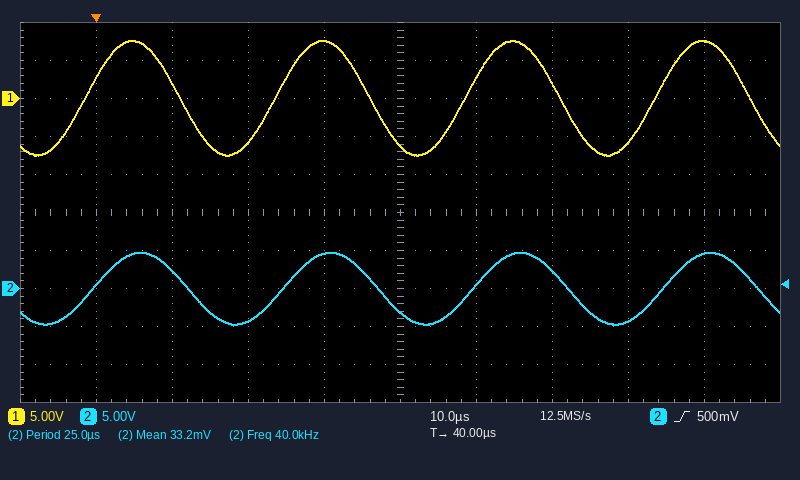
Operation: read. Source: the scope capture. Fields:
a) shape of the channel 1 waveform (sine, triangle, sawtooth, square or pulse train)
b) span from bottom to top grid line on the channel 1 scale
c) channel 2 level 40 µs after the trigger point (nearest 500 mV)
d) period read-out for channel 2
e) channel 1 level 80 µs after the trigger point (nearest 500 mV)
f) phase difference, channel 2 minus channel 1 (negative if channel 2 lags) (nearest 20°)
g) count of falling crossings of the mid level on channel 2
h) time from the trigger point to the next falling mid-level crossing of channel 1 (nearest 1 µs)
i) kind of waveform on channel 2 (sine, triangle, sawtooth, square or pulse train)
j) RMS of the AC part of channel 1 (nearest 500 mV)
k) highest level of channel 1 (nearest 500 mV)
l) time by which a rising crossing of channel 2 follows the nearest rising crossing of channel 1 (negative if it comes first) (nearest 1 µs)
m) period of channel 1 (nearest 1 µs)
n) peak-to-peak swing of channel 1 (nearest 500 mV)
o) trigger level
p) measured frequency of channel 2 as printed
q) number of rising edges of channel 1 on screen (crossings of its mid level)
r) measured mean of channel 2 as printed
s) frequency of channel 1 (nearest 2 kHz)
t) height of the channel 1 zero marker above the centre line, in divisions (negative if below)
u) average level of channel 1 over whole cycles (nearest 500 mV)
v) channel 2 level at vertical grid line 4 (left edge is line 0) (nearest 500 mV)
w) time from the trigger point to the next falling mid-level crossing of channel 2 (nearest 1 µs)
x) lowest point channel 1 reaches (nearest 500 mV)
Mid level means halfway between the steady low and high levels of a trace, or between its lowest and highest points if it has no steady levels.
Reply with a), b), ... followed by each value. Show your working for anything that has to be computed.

a) sine
b) 50 V
c) -3.0 V
d) 25.0 µs
e) 7.5 V
f) −360° × (+1 µs) / 25 µs ≈ -14.4°, so -20° to the nearest 20°
g) 4
h) 11 µs
i) sine
j) 15.0 V / (2√2) ≈ 5.30 V, so 5.5 V to the nearest 500 mV
k) 7.5 V
l) +1 µs
m) 25 µs
n) 7.5 V − (-7.5 V) = 15.0 V
o) 500 mV
p) 40.0 kHz
q) 4
r) 33.2 mV
s) 1 / 25 µs ≈ 40 kHz
t) +3.0 div
u) (7.5 V + (-7.5 V)) / 2 ≈ 0.0 V
v) 4.5 V
w) 12 µs
x) -7.5 V
